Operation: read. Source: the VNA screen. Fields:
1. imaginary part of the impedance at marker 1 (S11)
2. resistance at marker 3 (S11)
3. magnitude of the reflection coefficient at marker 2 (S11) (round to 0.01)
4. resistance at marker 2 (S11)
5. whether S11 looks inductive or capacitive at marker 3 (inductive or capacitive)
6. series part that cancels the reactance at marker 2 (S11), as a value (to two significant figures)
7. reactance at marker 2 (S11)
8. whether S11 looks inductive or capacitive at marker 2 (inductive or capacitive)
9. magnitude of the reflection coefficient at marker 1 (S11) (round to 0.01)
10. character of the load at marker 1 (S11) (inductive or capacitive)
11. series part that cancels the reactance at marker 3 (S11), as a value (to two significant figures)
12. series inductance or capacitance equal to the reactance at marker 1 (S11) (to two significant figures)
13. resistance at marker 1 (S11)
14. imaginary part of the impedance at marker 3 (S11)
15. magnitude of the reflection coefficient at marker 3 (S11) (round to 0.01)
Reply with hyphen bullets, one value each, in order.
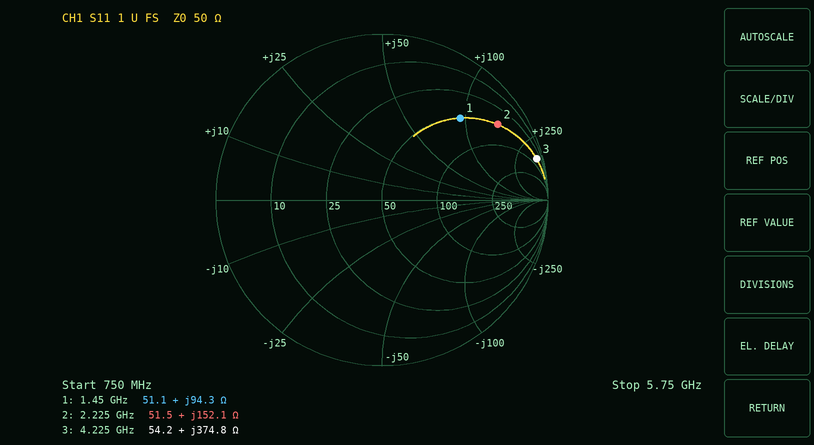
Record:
- +94.3 Ω
- 54.2 Ω
- 0.83
- 51.5 Ω
- inductive
- 470 fF
- +152.1 Ω
- inductive
- 0.68
- inductive
- 100 fF
- 10 nH
- 51.1 Ω
- +374.8 Ω
- 0.96
